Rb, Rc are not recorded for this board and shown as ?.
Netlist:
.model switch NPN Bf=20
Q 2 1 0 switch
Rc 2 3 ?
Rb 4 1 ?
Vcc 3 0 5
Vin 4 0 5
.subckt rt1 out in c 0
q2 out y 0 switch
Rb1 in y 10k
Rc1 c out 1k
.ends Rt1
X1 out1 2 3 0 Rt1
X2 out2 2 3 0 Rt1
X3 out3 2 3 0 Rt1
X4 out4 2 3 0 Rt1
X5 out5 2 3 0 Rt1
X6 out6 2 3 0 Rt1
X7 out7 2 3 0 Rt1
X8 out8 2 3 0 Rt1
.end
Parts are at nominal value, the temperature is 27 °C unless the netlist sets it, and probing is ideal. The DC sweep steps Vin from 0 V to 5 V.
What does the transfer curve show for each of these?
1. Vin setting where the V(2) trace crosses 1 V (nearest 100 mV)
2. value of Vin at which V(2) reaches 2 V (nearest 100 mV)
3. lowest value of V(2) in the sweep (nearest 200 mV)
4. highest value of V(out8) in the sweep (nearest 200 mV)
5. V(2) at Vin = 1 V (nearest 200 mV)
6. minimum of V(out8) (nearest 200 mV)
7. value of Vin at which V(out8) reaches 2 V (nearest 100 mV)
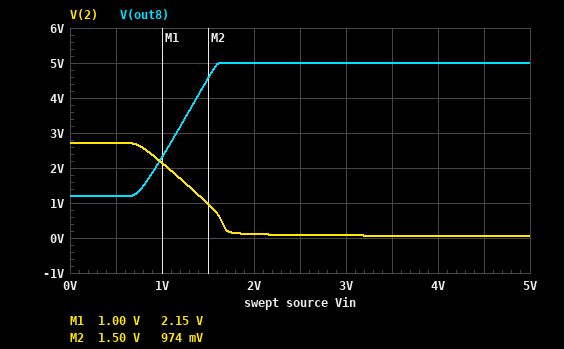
1.5 V
1.1 V
0 V
5.0 V
2.2 V
1.2 V
900 mV
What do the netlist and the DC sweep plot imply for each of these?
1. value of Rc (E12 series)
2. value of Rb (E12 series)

1.5 kΩ
5.6 kΩ
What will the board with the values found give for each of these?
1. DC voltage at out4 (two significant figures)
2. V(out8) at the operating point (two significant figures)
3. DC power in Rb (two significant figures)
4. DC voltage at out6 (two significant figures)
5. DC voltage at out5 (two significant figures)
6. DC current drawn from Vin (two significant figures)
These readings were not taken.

5.0 V
5.0 V
3.1 mW
5.0 V
5.0 V
750 µA
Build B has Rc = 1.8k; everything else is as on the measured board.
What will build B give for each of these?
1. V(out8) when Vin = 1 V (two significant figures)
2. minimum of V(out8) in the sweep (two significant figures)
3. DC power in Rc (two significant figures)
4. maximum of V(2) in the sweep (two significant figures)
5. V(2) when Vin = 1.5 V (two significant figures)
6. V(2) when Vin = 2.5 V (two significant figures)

2.8 V
1.6 V
14 mW
2.5 V
490 mV
78 mV
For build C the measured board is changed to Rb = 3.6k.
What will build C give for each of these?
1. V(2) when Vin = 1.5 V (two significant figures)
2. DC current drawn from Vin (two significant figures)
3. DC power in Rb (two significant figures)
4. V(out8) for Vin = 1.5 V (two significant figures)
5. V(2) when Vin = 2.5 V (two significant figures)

120 mV
1.2 mA
4.9 mW
5.0 V
68 mV
